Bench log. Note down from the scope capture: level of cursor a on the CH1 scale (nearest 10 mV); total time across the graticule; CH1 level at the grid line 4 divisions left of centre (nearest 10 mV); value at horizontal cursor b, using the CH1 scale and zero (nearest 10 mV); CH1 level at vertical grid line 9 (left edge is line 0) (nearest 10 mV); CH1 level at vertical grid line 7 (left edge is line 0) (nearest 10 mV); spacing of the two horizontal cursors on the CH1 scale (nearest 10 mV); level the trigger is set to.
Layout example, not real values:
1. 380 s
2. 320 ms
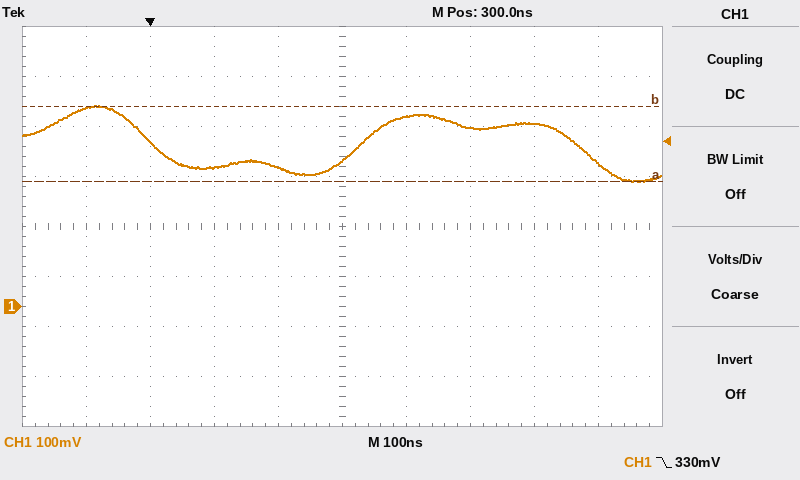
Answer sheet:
1. 250 mV
2. 1 µs
3. 400 mV
4. 400 mV
5. 290 mV
6. 360 mV
7. 150 mV
8. 330 mV
